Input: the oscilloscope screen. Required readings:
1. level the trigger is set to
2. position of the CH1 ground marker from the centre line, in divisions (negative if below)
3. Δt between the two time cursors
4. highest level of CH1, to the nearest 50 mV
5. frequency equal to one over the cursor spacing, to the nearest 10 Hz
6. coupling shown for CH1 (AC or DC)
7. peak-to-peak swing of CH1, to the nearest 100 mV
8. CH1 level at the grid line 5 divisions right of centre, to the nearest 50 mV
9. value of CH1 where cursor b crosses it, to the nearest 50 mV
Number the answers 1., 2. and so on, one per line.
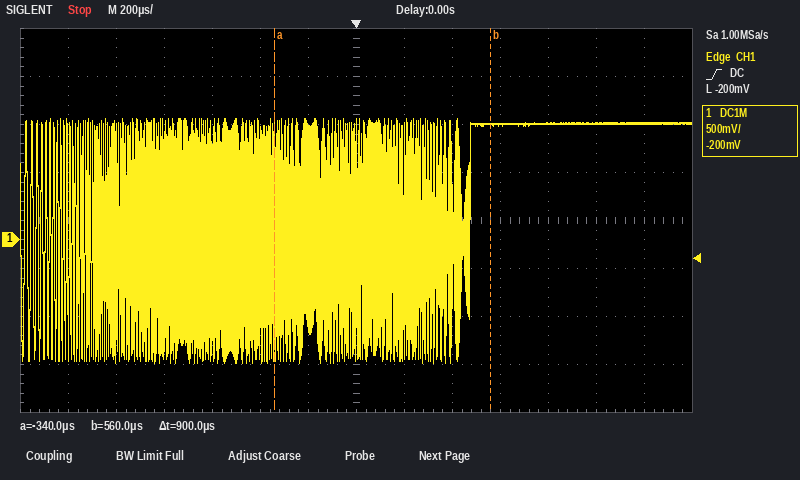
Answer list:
1. -200 mV
2. -0.4 div
3. 900 µs
4. 1.25 V
5. 1.11 kHz
6. DC
7. 2.50 V
8. 1.20 V
9. 1.20 V
